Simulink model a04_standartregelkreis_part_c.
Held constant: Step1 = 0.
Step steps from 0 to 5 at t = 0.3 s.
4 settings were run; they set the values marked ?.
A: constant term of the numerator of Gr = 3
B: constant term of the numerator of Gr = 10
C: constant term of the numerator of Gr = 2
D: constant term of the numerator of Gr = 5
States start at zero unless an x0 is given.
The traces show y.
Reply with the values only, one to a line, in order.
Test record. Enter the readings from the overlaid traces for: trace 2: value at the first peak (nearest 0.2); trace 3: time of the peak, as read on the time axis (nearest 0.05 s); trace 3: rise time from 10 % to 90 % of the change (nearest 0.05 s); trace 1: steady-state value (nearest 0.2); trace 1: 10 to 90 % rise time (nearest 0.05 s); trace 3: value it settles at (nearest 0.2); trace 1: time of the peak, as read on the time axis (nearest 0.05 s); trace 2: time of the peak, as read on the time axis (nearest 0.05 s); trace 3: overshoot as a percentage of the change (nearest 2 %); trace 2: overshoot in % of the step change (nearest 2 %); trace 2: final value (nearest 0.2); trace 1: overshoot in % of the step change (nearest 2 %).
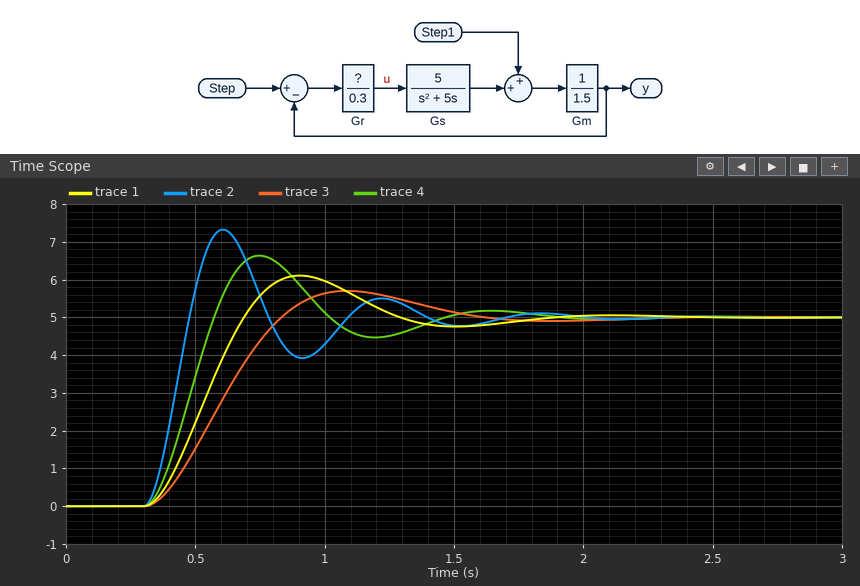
7.4
1.10 s
0.35 s
5.0
0.25 s
5.0
0.90 s
0.60 s
14 %
46 %
5.0
22 %
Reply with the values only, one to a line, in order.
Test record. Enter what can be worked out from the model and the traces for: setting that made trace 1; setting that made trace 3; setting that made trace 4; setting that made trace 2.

A
C
D
B
